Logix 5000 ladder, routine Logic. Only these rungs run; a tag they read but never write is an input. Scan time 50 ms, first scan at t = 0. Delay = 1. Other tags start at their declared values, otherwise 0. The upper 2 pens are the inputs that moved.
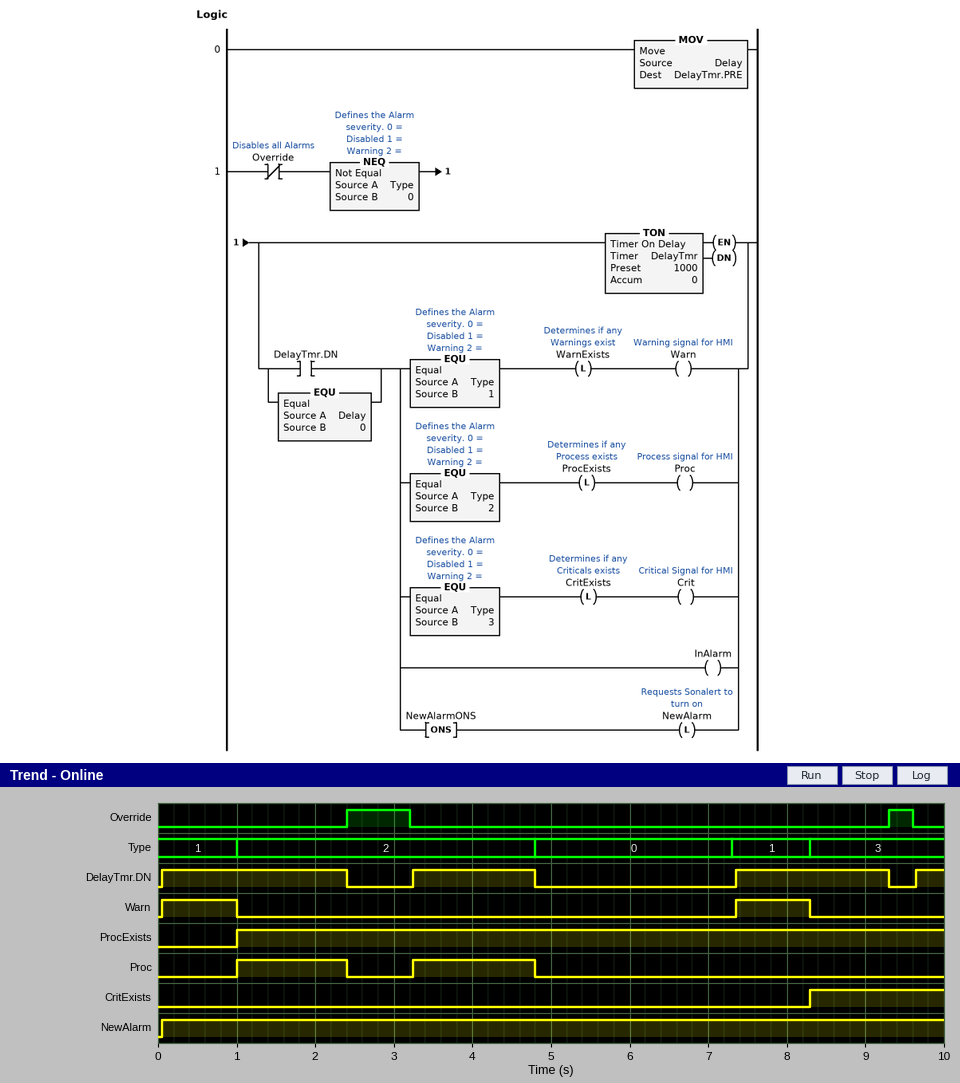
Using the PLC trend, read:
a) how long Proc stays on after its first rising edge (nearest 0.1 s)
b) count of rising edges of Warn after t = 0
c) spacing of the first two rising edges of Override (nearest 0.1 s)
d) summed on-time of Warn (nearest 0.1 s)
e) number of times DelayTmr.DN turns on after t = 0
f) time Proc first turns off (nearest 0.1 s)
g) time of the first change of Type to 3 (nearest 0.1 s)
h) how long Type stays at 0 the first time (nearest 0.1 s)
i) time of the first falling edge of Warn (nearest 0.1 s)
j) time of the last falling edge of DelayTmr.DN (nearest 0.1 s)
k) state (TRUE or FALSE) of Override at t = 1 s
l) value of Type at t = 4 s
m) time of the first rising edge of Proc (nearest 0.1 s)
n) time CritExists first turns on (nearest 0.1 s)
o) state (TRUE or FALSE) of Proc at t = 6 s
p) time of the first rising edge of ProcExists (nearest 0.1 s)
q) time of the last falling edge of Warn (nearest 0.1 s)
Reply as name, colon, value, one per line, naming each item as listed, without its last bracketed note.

how long Proc stays on after its first rising edge: 1.4 s
count of rising edges of Warn after t = 0: 2
spacing of the first two rising edges of Override: 6.9 s
summed on-time of Warn: 1.9 s
number of times DelayTmr.DN turns on after t = 0: 4
time Proc first turns off: 2.4 s
time of the first change of Type to 3: 8.3 s
how long Type stays at 0 the first time: 2.5 s
time of the first falling edge of Warn: 1.0 s
time of the last falling edge of DelayTmr.DN: 9.3 s
state (TRUE or FALSE) of Override at t = 1 s: FALSE
value of Type at t = 4 s: 2
time of the first rising edge of Proc: 1.0 s
time CritExists first turns on: 8.3 s
state (TRUE or FALSE) of Proc at t = 6 s: FALSE
time of the first rising edge of ProcExists: 1.0 s
time of the last falling edge of Warn: 8.3 s
